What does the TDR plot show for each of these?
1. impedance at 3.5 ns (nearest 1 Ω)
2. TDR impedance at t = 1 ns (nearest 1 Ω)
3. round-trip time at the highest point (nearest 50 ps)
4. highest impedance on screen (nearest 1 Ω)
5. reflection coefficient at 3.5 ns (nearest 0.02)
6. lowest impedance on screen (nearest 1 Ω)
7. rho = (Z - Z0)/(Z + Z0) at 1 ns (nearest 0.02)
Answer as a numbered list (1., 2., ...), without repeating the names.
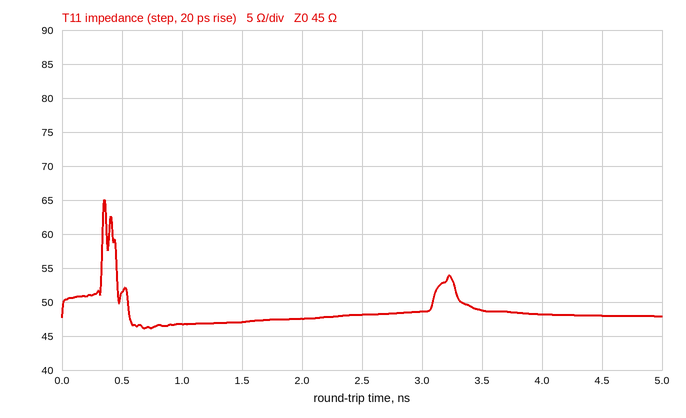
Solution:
1. 49 Ω
2. 47 Ω
3. 350 ps
4. 65 Ω
5. +0.04
6. 46 Ω
7. +0.02
